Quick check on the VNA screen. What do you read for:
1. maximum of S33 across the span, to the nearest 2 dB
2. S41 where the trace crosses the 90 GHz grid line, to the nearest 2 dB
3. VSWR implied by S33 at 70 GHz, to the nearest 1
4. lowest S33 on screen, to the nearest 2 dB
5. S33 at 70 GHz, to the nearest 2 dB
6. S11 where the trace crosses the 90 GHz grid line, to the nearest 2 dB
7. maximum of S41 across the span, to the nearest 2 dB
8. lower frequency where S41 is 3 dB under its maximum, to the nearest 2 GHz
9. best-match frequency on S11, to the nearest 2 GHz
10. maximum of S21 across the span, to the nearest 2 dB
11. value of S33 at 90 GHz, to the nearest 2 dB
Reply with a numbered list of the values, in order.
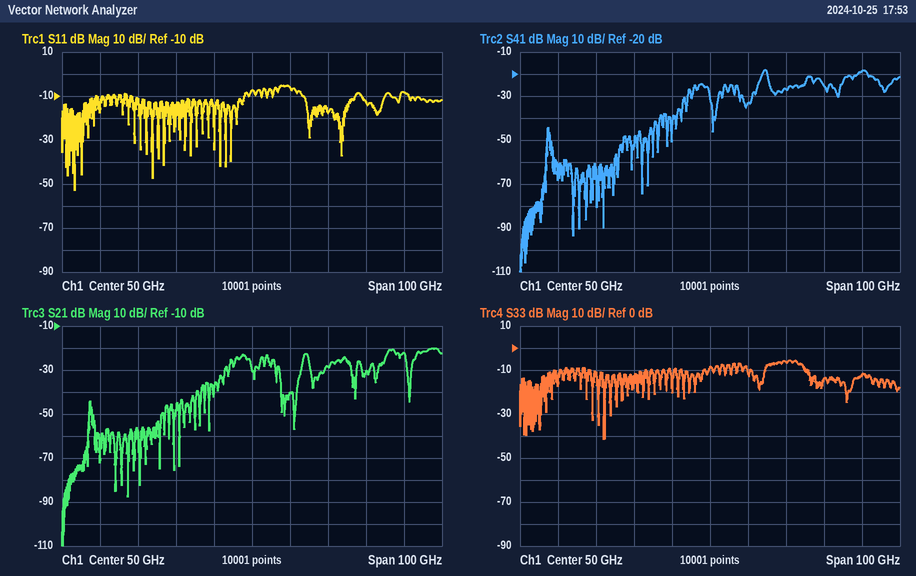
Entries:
1. -6 dB
2. -18 dB
3. 3
4. -42 dB
5. -6 dB
6. -8 dB
7. -18 dB
8. 64 GHz
9. 4 GHz
10. -20 dB
11. -12 dB
